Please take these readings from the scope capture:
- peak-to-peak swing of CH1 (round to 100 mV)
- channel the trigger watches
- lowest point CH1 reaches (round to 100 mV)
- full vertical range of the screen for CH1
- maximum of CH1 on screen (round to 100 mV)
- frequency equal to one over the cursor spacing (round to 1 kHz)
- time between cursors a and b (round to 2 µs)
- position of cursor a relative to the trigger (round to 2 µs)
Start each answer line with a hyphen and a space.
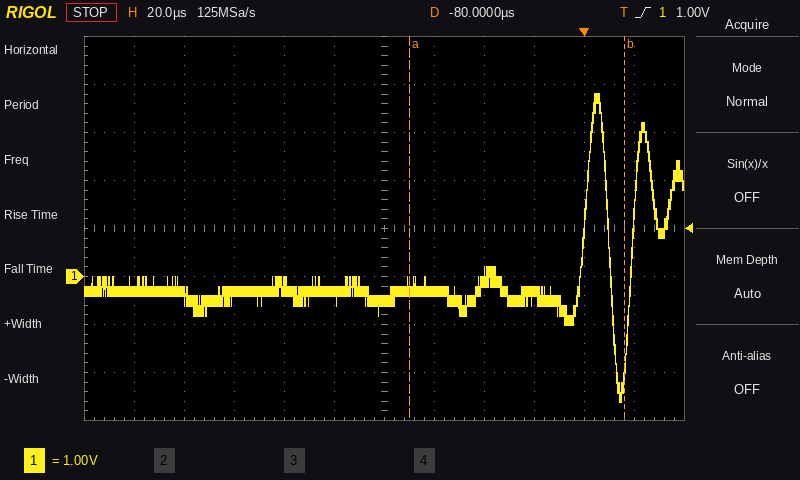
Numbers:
- 6.4 V
- CH1
- -2.6 V
- 8 V
- 3.8 V
- 12 kHz
- 86 µs
- -70 µs
